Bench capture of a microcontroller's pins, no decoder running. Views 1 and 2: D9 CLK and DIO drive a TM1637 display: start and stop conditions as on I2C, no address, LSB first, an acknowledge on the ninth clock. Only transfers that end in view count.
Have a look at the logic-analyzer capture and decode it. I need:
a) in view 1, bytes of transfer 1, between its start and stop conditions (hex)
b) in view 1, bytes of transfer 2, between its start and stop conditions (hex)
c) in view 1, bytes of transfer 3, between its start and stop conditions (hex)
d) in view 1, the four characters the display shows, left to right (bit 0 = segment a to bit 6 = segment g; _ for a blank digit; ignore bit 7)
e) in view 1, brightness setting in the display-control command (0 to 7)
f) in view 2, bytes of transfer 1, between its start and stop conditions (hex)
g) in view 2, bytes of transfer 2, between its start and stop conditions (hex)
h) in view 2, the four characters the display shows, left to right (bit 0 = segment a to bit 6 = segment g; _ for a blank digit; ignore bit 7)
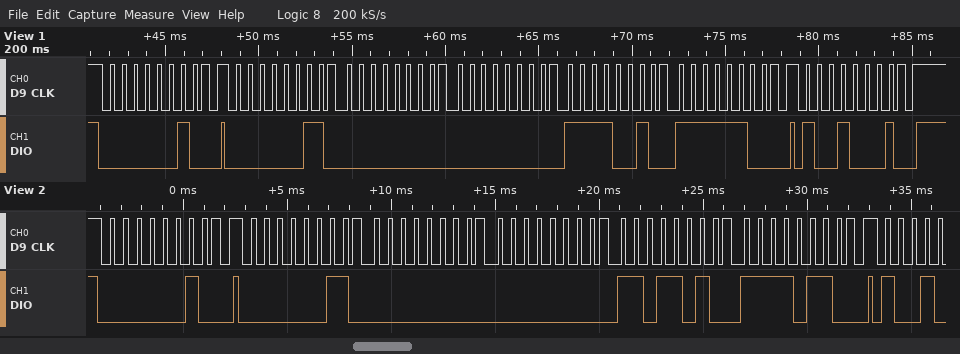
40
C0 00 00 4F 3F
89
__30
1
40
C0 00 00 5B 6F
__29
